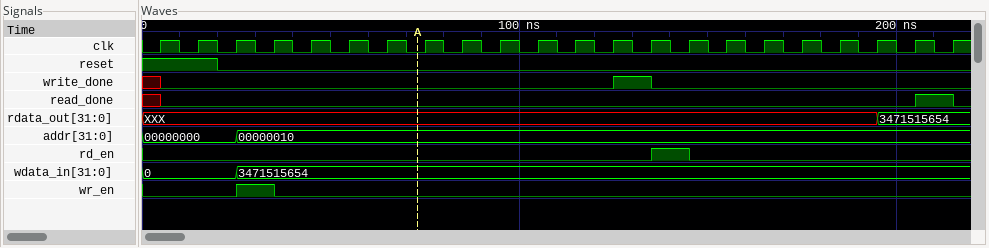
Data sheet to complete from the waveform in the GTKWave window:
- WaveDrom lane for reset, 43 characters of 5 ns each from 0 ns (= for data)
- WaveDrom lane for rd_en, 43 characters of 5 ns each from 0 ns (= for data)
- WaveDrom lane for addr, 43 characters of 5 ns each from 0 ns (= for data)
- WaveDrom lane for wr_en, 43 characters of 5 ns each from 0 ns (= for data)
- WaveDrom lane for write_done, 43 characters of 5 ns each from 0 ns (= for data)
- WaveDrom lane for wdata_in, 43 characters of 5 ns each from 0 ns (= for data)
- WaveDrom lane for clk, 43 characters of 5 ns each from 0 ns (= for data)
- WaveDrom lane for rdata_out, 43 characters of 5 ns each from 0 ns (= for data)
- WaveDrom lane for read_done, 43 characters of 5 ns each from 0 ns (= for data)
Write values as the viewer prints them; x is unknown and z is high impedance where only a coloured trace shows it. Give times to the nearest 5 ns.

{name: 'reset', wave: '1...0......................................'}
{name: 'rd_en', wave: '0..........................1.0.............'}
{name: 'addr', wave: '=....=.....................................', data: '00000000 00000010'}
{name: 'wr_en', wave: '0....1.0...................................'}
{name: 'write_done', wave: 'x0.......................1.0...............'}
{name: 'wdata_in', wave: '=....=.....................................', data: '0 3471515654'}
{name: 'clk', wave: '0101010101010101010101010101010101010101010'}
{name: 'rdata_out', wave: 'x......................................=...', data: '3471515654'}
{name: 'read_done', wave: 'x0.......................................1.'}
